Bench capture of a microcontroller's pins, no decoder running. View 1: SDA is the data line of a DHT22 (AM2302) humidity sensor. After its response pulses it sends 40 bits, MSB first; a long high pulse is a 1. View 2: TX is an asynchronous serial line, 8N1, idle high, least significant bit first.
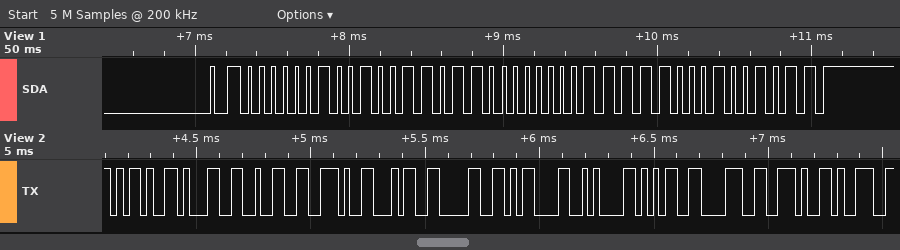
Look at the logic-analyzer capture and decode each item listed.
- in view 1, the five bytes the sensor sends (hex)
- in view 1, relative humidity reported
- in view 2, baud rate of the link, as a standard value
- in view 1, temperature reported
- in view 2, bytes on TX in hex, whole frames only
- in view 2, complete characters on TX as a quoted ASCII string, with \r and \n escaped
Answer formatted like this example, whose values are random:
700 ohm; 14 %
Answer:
02 4D 80 7C 4B; 58.9 %; 38400 baud; -12.4 °C; 2D 31 32 2E 34 30 0D 0A 35 38 2E 39; "-12.40\r\n58.9"
